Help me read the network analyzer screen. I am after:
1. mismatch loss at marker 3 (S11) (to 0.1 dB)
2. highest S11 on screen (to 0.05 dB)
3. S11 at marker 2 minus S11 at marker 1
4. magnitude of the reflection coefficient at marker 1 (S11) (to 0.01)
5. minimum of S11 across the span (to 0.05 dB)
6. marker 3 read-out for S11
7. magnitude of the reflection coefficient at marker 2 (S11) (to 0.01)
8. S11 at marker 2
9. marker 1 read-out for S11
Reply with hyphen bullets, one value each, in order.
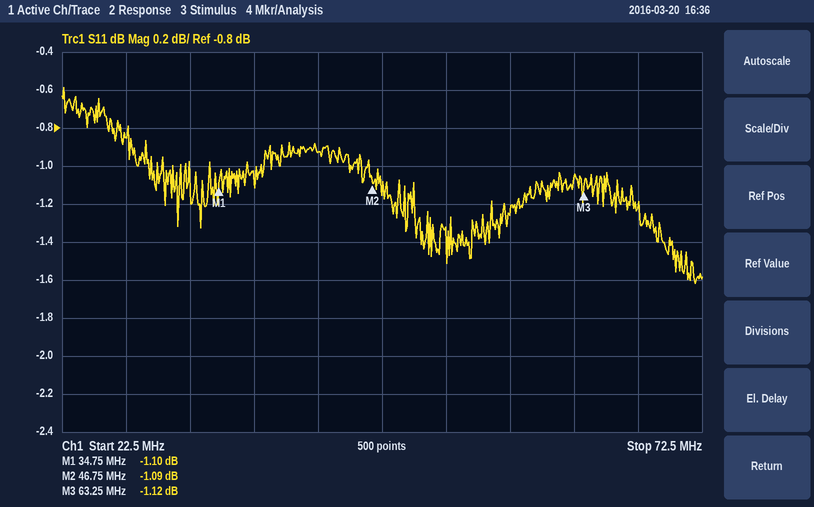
- 6.4 dB
- -0.60 dB
- 0.01 dB
- 0.88
- -1.60 dB
- -1.12 dB
- 0.88
- -1.09 dB
- -1.10 dB
